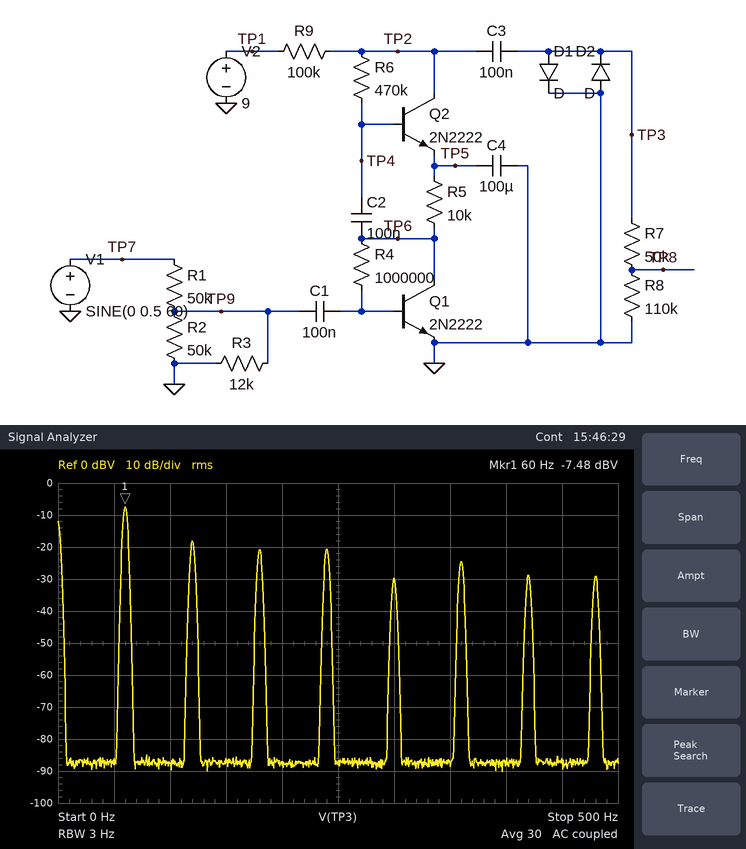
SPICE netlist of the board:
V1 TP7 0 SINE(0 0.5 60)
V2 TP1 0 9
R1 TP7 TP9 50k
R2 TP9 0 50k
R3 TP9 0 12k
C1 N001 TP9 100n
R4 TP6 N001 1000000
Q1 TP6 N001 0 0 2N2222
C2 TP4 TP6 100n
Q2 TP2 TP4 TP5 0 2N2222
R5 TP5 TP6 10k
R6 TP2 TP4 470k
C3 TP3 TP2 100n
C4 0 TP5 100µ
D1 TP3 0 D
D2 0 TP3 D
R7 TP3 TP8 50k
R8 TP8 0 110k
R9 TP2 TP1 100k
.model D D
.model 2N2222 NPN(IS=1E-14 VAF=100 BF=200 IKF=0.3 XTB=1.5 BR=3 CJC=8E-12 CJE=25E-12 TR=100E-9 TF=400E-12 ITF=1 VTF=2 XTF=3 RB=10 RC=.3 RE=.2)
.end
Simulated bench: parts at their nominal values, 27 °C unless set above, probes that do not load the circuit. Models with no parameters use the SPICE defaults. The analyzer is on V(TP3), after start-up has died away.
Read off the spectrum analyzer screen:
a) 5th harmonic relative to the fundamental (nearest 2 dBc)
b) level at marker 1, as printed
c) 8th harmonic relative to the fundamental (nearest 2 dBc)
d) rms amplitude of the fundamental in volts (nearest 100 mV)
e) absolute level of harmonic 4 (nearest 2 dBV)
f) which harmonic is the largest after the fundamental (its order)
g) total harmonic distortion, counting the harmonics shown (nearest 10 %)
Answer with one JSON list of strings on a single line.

["-22 dBc", "-7.48 dBV", "-22 dBc", "400 mV", "-20 dBV", "2", "50 %"]
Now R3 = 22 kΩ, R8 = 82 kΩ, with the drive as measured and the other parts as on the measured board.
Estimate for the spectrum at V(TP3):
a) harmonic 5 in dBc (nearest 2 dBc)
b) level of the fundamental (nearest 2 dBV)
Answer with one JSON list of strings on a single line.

["-18 dBc", "-8 dBV"]
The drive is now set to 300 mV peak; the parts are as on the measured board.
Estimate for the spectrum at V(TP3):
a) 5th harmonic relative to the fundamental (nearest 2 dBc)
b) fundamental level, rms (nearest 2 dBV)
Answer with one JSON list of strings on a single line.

["-26 dBc", "-8 dBV"]
